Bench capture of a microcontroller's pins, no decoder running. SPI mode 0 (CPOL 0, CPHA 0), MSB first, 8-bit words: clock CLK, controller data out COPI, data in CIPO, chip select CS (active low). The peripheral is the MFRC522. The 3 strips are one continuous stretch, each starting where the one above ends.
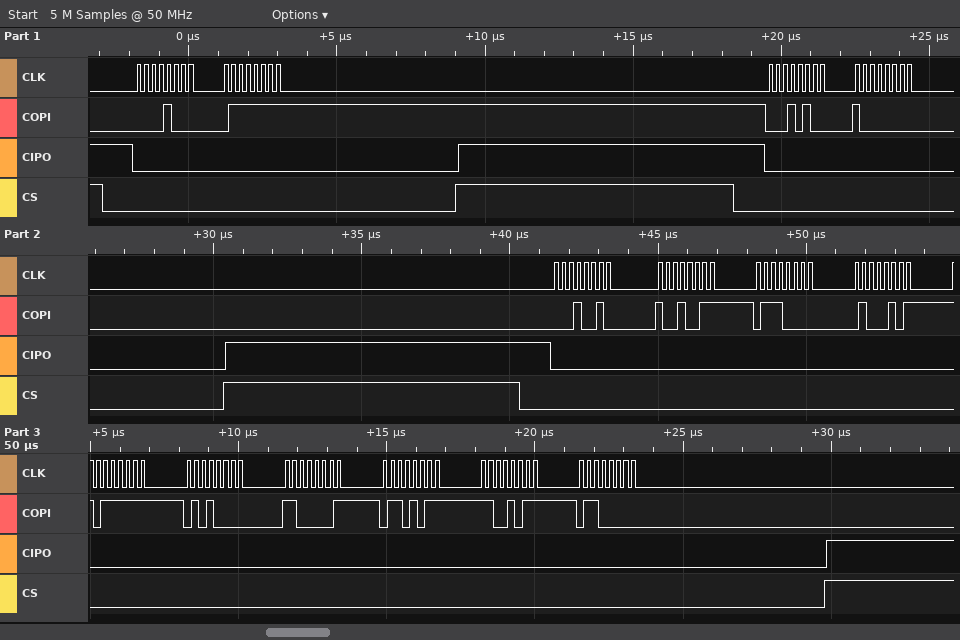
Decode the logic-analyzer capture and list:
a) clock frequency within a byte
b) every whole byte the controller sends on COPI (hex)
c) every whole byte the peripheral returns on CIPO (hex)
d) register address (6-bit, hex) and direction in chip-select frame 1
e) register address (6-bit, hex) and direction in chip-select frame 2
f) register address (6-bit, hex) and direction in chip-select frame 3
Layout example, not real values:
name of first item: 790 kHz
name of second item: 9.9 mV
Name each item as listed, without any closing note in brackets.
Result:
clock frequency within a byte: 4 MHz
every whole byte the controller sends on COPI: 08 7F 14 80 12 93 70 45 BF 50 C1 6B CB 60
every whole byte the peripheral returns on CIPO: 00 00 00 00 00 00 00 00 00 00 00 00 00 00
register address (6-bit, hex) and direction in chip-select frame 1: 0x04 write
register address (6-bit, hex) and direction in chip-select frame 2: 0x0A write
register address (6-bit, hex) and direction in chip-select frame 3: 0x09 write
